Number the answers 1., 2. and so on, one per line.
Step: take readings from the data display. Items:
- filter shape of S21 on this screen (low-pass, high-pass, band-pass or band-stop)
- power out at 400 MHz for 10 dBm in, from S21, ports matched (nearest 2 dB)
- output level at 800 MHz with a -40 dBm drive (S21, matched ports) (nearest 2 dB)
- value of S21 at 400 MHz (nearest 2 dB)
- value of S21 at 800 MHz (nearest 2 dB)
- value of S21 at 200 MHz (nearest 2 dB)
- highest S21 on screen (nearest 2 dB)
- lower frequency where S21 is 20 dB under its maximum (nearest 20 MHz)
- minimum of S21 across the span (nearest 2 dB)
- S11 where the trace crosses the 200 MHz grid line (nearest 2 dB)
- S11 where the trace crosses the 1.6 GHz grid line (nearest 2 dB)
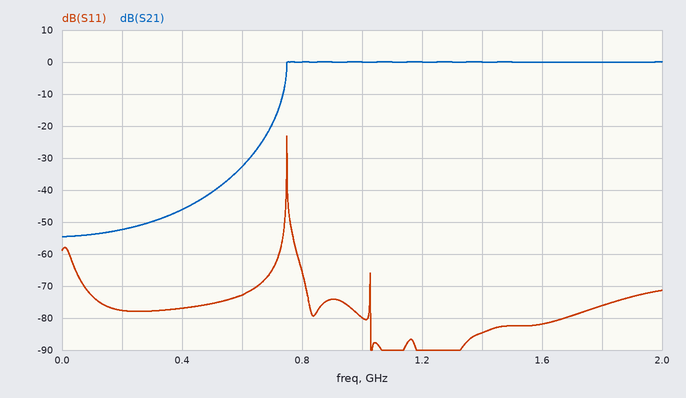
1. high-pass
2. -36 dBm
3. -40 dBm
4. -46 dB
5. 0 dB
6. -52 dB
7. 0 dB
8. 700 MHz
9. -54 dB
10. -78 dB
11. -82 dB
